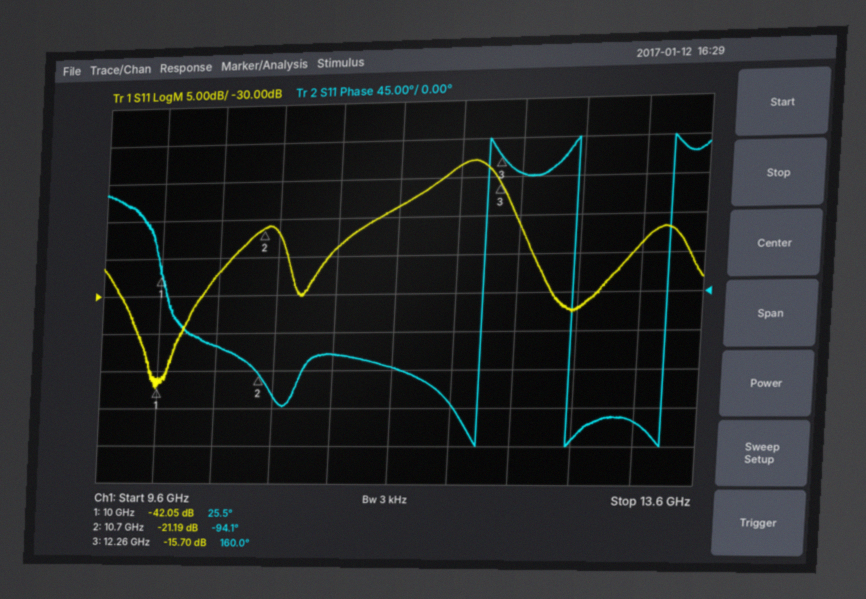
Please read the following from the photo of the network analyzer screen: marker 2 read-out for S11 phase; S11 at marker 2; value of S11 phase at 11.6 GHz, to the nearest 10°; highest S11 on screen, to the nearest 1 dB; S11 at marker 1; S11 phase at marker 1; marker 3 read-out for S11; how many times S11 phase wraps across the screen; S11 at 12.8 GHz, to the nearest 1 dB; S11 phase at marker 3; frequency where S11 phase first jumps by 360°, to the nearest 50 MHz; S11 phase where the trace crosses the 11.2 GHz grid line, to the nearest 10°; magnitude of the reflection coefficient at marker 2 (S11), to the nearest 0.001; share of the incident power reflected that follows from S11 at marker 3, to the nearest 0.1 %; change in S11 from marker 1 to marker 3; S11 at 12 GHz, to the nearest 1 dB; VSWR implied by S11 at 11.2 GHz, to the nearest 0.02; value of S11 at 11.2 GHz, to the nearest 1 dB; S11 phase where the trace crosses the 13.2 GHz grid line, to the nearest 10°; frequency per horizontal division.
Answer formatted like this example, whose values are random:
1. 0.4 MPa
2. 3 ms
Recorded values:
1. -94.1°
2. -21.19 dB
3. -90°
4. -13 dB
5. -42.05 dB
6. 25.5°
7. -15.70 dB
8. 3
9. -32 dB
10. 160.0°
11. 12.20 GHz
12. -70°
13. 0.087
14. 2.7 %
15. 26.35 dB
16. -13 dB
17. 1.14
18. -24 dB
19. -150°
20. 400 MHz
